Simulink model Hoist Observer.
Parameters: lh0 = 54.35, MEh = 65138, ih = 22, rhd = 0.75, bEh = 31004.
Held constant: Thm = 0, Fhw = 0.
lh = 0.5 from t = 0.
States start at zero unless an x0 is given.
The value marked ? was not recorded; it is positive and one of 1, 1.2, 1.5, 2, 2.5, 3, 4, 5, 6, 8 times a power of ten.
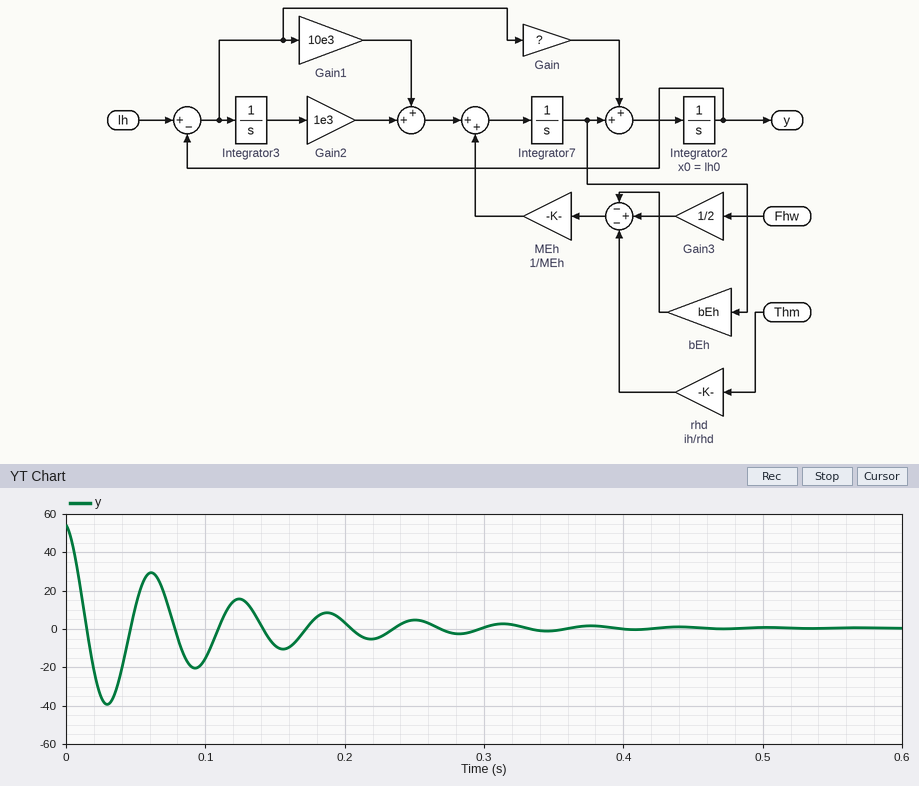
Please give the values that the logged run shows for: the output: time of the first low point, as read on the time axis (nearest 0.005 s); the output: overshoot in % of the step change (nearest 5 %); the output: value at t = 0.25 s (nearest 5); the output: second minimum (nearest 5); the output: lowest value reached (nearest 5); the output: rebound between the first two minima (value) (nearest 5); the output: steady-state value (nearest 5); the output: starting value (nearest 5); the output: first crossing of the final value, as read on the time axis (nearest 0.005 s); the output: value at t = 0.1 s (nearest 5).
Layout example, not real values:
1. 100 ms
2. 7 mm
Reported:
1. 0.030 s
2. 75 %
3. 5
4. -20
5. -40
6. 30
7. 0
8. 55
9. 0.015 s
10. -15
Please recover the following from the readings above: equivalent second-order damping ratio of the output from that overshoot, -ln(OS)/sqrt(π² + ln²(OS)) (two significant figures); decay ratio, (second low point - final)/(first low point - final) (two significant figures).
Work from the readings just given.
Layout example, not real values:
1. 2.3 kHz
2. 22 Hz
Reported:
1. 0.091
2. 0.50
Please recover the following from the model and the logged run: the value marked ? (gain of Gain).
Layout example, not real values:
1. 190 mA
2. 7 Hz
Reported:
1. 20
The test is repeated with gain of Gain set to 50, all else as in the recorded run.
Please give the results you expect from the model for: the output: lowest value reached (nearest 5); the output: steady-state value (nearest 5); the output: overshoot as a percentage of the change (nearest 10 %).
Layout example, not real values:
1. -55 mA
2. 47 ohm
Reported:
1. -25
2. 0
3. 50 %
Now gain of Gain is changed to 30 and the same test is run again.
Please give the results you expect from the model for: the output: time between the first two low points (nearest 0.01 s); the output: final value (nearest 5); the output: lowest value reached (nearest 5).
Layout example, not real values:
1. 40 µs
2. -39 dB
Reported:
1. 0.06 s
2. 0
3. -35
